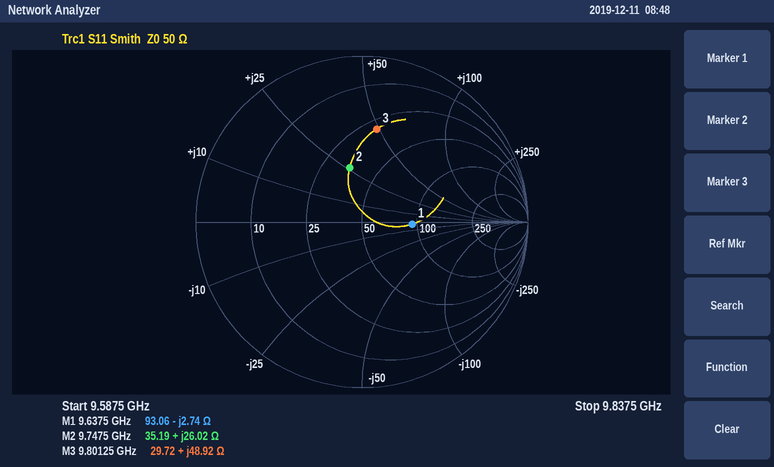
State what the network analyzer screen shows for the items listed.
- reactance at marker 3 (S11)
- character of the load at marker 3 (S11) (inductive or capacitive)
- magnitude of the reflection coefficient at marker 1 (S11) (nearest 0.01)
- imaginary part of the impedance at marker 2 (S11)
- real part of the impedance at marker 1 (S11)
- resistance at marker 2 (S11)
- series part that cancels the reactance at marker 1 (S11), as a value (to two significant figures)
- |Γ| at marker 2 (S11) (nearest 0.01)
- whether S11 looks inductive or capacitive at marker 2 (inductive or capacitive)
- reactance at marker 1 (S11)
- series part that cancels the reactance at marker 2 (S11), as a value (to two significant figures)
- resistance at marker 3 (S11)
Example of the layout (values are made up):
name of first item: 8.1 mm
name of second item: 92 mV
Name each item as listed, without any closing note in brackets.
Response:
reactance at marker 3: +48.92 Ω
character of the load at marker 3 (S11): inductive
magnitude of the reflection coefficient at marker 1 (S11): 0.30
imaginary part of the impedance at marker 2: +26.02 Ω
real part of the impedance at marker 1: 93.06 Ω
resistance at marker 2: 35.19 Ω
series part that cancels the reactance at marker 1 (S11), as a value: 45 pH
|Γ| at marker 2 (S11): 0.34
whether S11 looks inductive or capacitive at marker 2: inductive
reactance at marker 1: -2.74 Ω
series part that cancels the reactance at marker 2 (S11), as a value: 630 fF
resistance at marker 3: 29.72 Ω
